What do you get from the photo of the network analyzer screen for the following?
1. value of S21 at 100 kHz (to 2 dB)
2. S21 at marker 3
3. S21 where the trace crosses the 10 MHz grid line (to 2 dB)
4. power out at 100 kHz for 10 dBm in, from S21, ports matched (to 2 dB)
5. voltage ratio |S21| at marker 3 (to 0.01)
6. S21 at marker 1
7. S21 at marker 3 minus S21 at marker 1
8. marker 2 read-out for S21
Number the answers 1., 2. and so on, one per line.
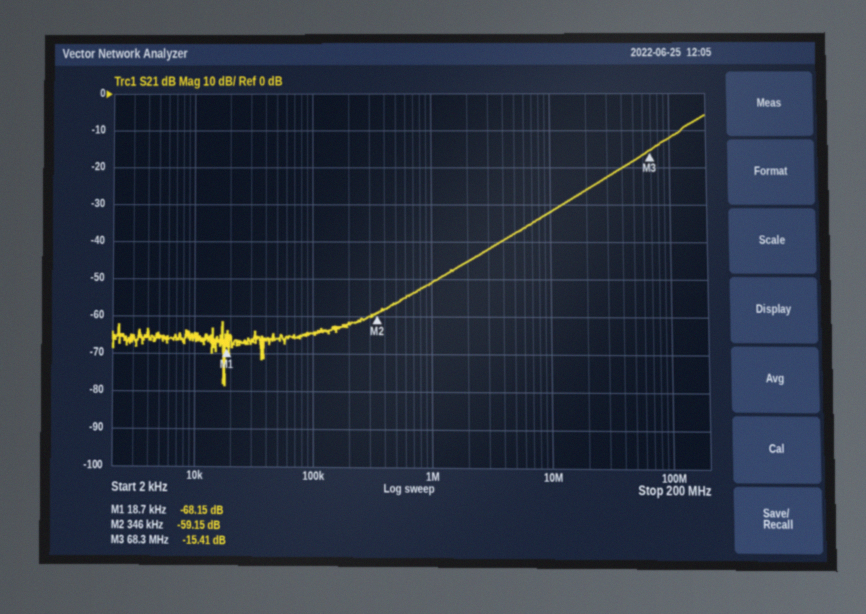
1. -64 dB
2. -15.41 dB
3. -32 dB
4. -54 dBm
5. 0.17
6. -68.15 dB
7. 52.74 dB
8. -59.15 dB
